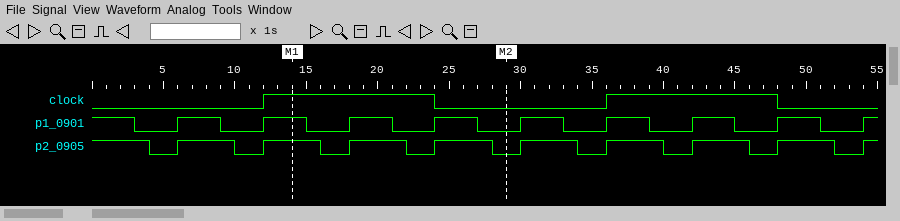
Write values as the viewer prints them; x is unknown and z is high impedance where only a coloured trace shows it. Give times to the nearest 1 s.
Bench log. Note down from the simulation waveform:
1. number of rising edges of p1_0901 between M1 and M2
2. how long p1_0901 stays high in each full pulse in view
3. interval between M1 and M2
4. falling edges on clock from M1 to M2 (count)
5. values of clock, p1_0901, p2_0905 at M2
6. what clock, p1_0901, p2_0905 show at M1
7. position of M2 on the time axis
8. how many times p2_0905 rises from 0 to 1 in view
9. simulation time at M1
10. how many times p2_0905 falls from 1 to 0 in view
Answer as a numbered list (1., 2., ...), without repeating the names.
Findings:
1. 2
2. 3 s, 3 s, 3 s, 3 s, 3 s, 3 s, 3 s, 3 s
3. 15 s
4. 1
5. clock=0, p1_0901=0, p2_0905=0
6. clock=1, p1_0901=1, p2_0905=1
7. 29 s
8. 9
9. 14 s
10. 9
